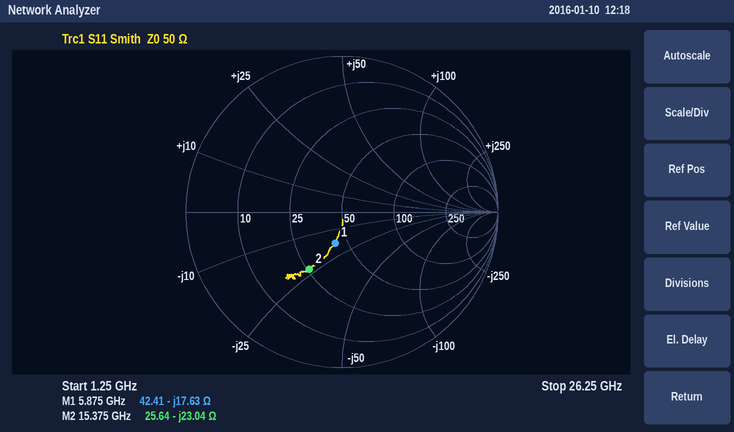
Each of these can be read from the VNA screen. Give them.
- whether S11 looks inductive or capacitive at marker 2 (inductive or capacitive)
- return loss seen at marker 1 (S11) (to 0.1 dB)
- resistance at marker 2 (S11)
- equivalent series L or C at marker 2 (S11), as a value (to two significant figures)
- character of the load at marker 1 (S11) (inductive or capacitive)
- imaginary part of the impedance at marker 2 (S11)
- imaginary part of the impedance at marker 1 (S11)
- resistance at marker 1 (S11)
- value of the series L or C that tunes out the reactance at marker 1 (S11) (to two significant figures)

capacitive
13.8 dB
25.64 Ω
450 fF
capacitive
-23.04 Ω
-17.63 Ω
42.41 Ω
480 pH
